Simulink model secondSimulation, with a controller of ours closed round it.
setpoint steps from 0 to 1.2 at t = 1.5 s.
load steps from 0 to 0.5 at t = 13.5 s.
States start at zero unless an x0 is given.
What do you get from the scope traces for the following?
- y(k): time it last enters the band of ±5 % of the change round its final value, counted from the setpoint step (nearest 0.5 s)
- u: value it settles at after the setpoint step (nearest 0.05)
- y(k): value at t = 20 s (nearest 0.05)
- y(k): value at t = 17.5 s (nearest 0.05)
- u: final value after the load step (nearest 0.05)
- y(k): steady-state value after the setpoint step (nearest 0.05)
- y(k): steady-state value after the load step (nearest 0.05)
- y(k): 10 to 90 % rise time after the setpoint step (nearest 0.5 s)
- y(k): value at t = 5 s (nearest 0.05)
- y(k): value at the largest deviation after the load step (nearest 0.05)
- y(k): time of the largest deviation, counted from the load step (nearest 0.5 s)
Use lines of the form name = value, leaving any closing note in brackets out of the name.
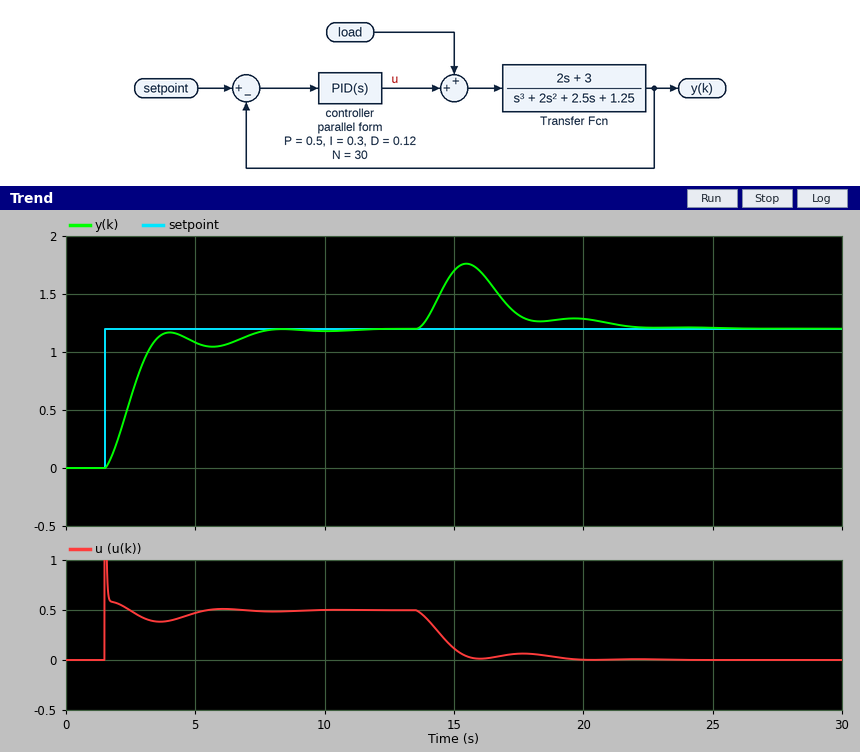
y(k): time it last enters the band of ±5 % of the change round its final value, counted from the setpoint step = 5.5 s
u: value it settles at after the setpoint step = 0.50
y(k): value at t = 20 s = 1.30
y(k): value at t = 17.5 s = 1.30
u: final value after the load step = 0.00
y(k): steady-state value after the setpoint step = 1.20
y(k): steady-state value after the load step = 1.20
y(k): 10 to 90 % rise time after the setpoint step = 1.5 s
y(k): value at t = 5 s = 1.10
y(k): value at the largest deviation after the load step = 1.75
y(k): time of the largest deviation, counted from the load step = 2.0 s
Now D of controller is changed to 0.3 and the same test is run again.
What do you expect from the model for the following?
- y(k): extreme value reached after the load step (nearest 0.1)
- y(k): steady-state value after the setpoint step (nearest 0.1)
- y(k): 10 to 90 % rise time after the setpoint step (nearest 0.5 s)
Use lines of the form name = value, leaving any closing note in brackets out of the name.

y(k): extreme value reached after the load step = 1.7
y(k): steady-state value after the setpoint step = 1.2
y(k): 10 to 90 % rise time after the setpoint step = 4.0 s
